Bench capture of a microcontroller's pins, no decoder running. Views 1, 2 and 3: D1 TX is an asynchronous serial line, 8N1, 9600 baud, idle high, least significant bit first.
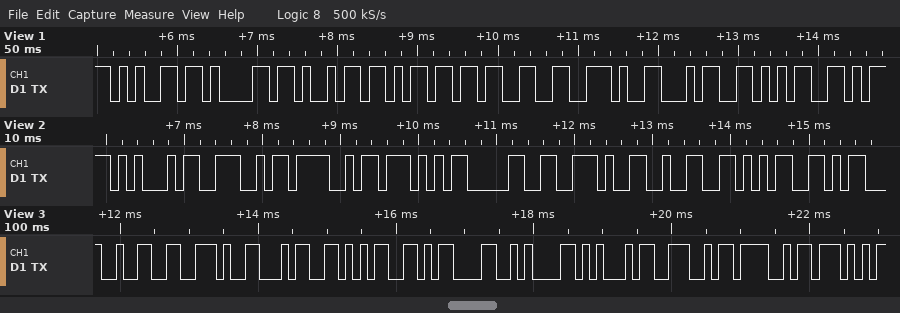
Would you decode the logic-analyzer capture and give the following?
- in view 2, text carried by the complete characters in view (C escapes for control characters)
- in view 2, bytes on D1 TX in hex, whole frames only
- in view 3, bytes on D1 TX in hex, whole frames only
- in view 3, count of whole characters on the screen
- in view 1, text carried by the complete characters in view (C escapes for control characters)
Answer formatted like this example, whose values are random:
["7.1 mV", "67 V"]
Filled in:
["\"ENOW0.25\"", "45 4E 4F 57 30 2E 32 35", "0x32 0x2E 0x34 0x35 0x0D 0x0A 0x45 0x4E 0x4F 0x57", "10", "\"eaim3.45\""]
